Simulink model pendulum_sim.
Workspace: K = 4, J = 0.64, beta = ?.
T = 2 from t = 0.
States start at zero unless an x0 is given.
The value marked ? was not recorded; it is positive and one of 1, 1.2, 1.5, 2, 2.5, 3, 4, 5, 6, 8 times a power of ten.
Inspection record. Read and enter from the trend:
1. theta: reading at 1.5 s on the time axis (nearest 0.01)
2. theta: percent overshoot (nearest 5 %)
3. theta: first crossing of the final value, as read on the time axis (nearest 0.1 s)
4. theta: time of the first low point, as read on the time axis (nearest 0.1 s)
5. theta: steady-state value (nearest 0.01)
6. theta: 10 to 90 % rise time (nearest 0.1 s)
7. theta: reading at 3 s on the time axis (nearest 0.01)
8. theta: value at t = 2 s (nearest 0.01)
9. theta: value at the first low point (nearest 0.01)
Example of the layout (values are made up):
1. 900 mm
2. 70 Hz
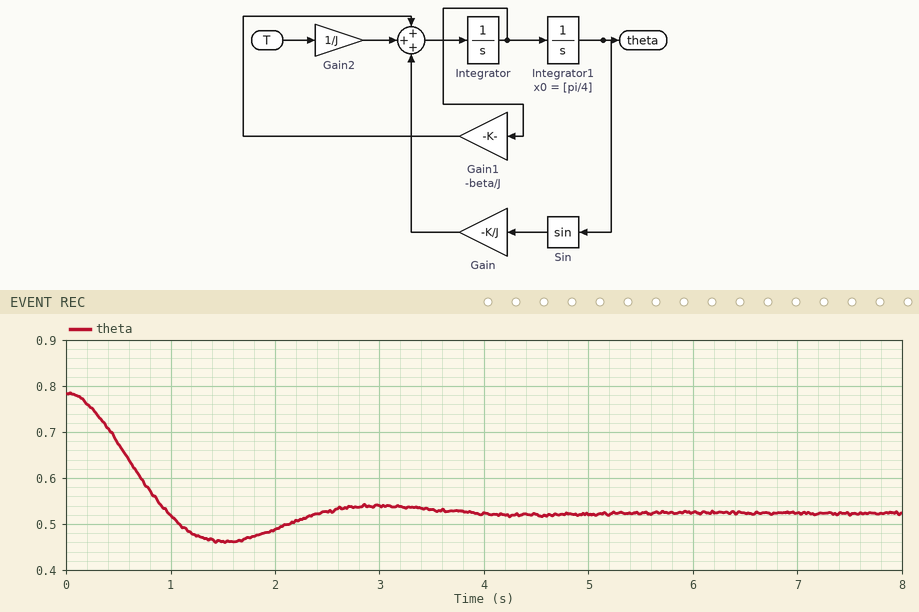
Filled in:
1. 0.46
2. 25 %
3. 1.0 s
4. 1.5 s
5. 0.52
6. 0.7 s
7. 0.54
8. 0.49
9. 0.46
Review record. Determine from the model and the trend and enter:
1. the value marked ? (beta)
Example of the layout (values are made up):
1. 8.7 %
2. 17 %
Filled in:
1. 1.2
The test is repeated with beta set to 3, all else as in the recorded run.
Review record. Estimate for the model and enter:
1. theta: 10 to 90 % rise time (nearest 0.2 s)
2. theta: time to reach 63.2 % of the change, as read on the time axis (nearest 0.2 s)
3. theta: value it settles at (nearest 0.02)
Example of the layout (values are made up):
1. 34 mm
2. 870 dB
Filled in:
1. 1.6 s
2. 1.0 s
3. 0.52
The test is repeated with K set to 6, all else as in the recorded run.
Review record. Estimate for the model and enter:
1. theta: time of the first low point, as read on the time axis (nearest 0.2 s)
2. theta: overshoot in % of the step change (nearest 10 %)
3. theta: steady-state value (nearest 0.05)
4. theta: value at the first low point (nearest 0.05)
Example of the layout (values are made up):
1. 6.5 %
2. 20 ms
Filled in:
1. 1.2 s
2. 30 %
3. 0.35
4. 0.20
